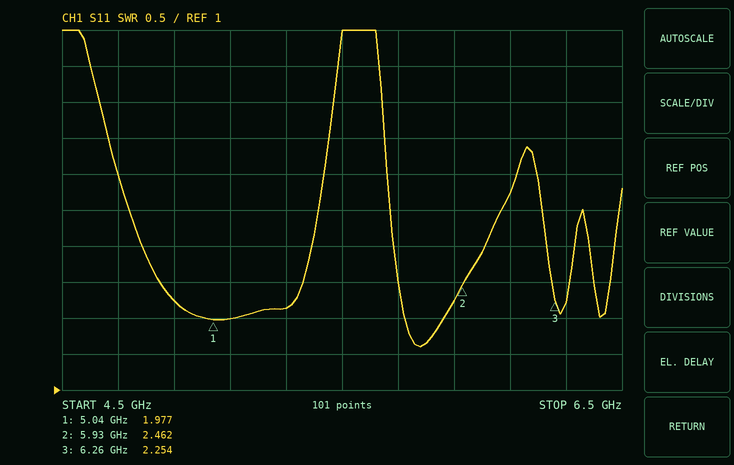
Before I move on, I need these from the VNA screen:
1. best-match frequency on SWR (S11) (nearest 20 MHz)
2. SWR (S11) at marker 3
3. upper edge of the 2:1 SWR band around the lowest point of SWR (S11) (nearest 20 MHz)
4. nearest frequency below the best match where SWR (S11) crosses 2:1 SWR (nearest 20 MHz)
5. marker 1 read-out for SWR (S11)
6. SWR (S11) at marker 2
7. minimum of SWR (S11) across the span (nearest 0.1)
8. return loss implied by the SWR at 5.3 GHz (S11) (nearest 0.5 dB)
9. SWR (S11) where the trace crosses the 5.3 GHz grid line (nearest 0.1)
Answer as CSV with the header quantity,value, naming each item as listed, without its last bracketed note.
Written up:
quantity,value
best-match frequency on SWR (S11),5.78 GHz
SWR (S11) at marker 3,2.254
upper edge of the 2:1 SWR band around the lowest point of SWR (S11),5.86 GHz
nearest frequency below the best match where SWR (S11) crosses 2:1 SWR,5.72 GHz
marker 1 read-out for SWR,1.977
SWR (S11) at marker 2,2.462
minimum of SWR (S11) across the span,1.6
return loss implied by the SWR at 5.3 GHz (S11),9.0 dB
SWR (S11) where the trace crosses the 5.3 GHz grid line,2.1
